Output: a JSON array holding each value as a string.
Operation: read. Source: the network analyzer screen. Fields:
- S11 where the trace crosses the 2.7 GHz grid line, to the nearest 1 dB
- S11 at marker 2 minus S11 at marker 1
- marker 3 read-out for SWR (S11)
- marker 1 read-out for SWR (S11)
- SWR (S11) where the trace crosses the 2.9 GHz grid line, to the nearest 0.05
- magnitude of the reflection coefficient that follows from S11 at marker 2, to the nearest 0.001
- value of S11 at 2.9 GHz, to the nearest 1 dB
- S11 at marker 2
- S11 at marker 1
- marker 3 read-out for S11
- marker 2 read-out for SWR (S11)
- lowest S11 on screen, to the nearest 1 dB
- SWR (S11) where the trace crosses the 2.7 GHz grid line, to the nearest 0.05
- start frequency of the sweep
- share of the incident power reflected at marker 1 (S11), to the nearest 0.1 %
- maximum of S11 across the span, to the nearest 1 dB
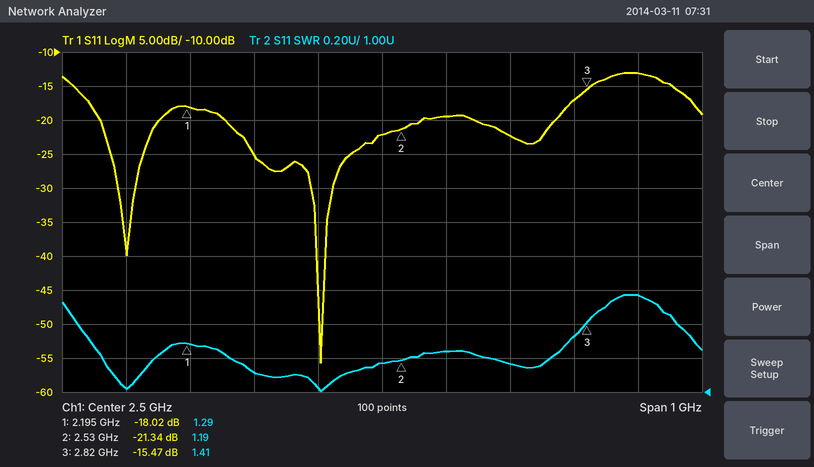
["-22 dB", "-3.32 dB", "1.41", "1.29", "1.55", "0.086", "-13 dB", "-21.34 dB", "-18.02 dB", "-15.47 dB", "1.19", "-56 dB", "1.15", "2 GHz", "1.6 %", "-13 dB"]
